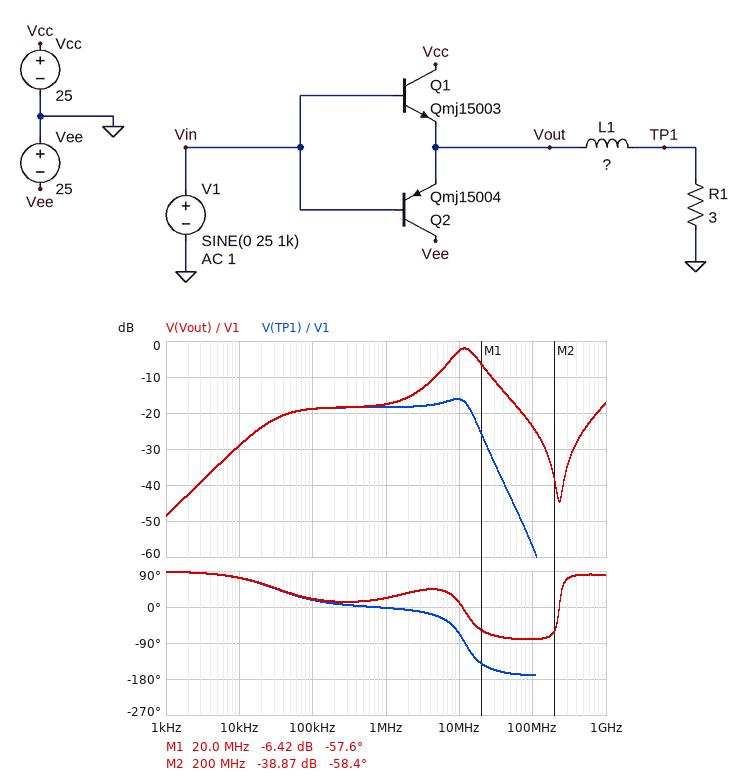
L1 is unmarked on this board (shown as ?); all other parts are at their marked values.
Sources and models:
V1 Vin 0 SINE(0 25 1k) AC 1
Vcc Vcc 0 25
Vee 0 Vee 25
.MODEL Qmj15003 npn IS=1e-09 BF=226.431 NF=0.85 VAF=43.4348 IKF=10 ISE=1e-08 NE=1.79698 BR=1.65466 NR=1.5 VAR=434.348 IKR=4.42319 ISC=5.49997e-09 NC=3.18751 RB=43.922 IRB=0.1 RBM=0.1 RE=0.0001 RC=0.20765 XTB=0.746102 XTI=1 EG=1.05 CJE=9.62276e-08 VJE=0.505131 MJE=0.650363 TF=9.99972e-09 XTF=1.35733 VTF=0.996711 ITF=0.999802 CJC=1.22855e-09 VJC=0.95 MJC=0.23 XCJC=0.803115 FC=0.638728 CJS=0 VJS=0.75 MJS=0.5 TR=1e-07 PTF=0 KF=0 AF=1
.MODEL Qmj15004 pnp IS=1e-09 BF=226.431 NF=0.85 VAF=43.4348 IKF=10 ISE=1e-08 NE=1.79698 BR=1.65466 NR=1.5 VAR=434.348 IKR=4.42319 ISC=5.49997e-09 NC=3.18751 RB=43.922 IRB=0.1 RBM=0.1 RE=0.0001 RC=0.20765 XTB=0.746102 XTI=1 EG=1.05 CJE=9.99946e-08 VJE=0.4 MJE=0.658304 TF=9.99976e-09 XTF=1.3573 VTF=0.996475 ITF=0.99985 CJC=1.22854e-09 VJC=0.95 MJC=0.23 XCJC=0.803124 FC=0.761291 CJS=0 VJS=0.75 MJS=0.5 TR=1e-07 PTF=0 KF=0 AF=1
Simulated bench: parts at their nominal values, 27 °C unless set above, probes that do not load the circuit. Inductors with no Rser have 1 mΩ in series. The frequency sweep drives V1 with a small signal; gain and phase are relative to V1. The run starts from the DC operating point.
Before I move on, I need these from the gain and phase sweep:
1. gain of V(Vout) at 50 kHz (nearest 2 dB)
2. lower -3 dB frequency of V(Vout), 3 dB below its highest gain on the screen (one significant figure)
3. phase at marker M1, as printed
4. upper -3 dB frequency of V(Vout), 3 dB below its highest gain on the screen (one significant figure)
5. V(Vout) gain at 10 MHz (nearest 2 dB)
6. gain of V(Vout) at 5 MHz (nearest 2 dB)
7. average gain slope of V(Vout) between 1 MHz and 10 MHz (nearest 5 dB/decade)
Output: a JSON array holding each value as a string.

["-20 dB", "8 MHz", "-57.6 deg", "20 MHz", "-2 dB", "-10 dB", "15 dB/decade"]
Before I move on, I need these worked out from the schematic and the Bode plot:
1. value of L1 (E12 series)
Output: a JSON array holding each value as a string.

["220 nH"]
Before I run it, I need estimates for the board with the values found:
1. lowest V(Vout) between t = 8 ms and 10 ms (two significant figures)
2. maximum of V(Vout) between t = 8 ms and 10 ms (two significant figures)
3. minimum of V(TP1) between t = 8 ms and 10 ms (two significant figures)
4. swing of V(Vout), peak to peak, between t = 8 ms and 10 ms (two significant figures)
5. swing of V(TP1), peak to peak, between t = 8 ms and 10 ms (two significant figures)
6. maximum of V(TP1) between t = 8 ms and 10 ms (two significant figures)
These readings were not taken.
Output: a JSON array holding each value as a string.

["-23 V", "23 V", "-23 V", "46 V", "46 V", "23 V"]
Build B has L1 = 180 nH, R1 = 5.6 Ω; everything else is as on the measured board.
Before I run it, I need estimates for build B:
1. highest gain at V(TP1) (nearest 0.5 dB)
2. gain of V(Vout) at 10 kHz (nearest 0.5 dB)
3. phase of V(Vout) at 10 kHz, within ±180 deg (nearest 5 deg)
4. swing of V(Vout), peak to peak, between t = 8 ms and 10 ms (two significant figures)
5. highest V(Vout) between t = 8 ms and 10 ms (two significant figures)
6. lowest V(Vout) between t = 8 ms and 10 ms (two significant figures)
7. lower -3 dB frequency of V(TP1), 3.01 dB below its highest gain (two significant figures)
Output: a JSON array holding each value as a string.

["-12.0 dB", "-23.5 dB", "70 deg", "47 V", "24 V", "-24 V", "49 kHz"]
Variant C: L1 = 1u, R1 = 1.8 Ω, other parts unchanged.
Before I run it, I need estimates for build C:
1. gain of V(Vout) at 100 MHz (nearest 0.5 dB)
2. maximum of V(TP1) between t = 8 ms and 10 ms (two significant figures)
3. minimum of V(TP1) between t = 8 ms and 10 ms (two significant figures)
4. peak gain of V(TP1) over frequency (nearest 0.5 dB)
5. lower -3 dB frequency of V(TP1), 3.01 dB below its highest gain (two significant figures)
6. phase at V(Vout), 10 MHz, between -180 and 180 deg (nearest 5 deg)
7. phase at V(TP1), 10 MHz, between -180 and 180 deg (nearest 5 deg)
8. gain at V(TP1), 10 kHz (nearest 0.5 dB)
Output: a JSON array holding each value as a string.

["-24.0 dB", "22 V", "-22 V", "-22.5 dB", "34 kHz", "-40 deg", "-130 deg", "-33.5 dB"]
